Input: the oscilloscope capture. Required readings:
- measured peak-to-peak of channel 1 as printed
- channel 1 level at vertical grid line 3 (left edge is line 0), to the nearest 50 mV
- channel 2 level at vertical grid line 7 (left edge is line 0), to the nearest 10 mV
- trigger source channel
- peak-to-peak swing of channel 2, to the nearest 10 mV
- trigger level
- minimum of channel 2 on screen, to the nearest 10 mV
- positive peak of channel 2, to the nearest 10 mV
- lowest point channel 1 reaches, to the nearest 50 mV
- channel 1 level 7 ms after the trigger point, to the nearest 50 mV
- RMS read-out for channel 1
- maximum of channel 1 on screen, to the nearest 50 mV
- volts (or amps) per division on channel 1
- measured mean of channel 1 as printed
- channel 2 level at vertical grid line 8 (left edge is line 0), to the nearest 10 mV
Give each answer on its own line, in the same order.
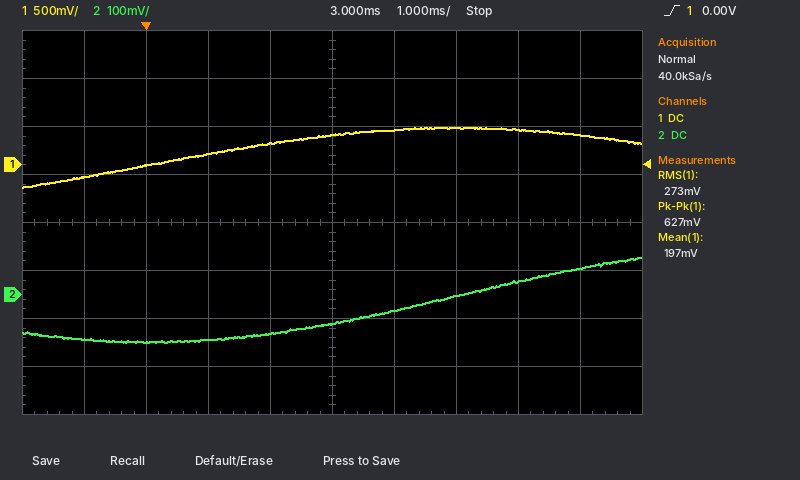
627 mV
100 mV
0 mV
channel 1
180 mV
0.00 V
-100 mV
80 mV
-250 mV
300 mV
273 mV
400 mV
500 mV
197 mV
30 mV
